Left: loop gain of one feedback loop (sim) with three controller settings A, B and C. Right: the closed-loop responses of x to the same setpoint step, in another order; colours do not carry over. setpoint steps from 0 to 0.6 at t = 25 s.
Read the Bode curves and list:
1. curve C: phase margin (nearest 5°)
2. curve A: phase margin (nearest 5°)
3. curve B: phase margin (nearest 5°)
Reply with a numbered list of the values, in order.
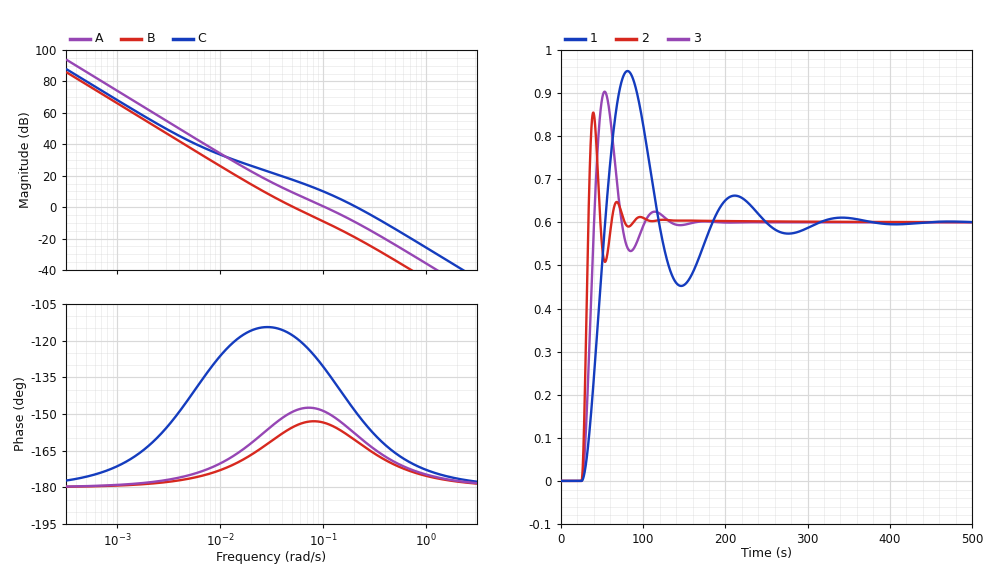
1. 30°
2. 30°
3. 25°
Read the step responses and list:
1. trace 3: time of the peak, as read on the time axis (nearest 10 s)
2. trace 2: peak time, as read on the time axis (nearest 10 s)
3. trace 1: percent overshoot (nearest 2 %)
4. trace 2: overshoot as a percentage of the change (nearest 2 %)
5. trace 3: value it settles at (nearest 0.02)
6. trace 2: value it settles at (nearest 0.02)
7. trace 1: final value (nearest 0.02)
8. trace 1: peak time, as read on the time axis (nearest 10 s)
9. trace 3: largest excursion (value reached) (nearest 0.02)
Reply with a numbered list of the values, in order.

1. 50 s
2. 40 s
3. 58 %
4. 42 %
5. 0.60
6. 0.60
7. 0.60
8. 80 s
9. 0.90
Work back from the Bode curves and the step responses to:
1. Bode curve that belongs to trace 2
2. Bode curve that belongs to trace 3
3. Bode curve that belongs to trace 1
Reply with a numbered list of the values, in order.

1. C
2. A
3. B
